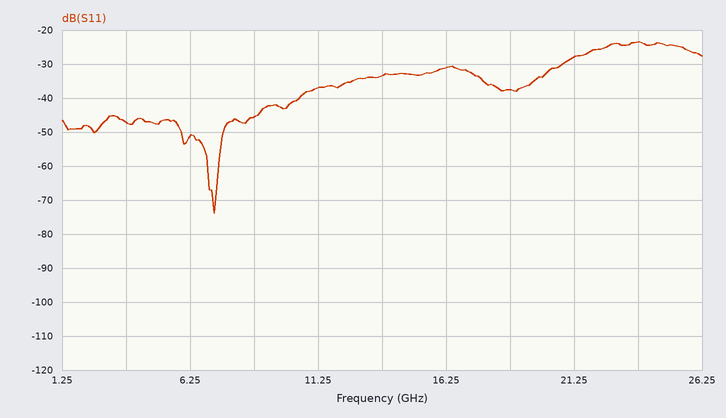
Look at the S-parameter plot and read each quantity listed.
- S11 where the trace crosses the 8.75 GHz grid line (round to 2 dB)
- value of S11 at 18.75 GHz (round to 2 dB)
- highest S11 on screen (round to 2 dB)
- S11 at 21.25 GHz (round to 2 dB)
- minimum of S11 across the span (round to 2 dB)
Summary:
-46 dB
-38 dB
-24 dB
-28 dB
-74 dB
